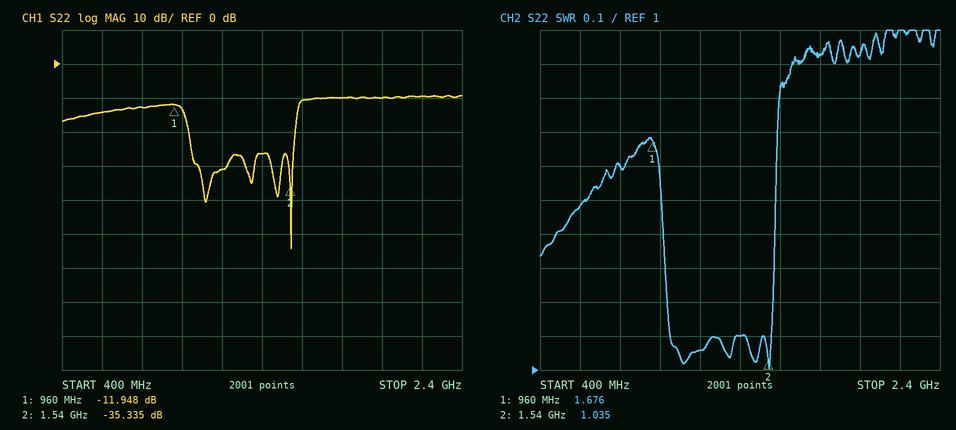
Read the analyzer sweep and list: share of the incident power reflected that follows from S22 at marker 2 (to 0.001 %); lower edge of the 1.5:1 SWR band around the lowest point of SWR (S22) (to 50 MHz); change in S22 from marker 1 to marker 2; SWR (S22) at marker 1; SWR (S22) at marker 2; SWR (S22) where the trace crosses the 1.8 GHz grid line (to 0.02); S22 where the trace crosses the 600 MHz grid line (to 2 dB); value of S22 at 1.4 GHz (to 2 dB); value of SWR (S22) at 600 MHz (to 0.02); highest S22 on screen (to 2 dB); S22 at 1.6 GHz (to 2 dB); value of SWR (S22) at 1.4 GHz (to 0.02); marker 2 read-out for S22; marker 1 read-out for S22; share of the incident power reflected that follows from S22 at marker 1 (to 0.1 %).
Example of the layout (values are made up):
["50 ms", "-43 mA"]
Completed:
["0.029 %", "1.00 GHz", "-23.387 dB", "1.676", "1.035", "1.92", "-14 dB", "-26 dB", "1.48", "-10 dB", "-10 dB", "1.10", "-35.335 dB", "-11.948 dB", "6.4 %"]
